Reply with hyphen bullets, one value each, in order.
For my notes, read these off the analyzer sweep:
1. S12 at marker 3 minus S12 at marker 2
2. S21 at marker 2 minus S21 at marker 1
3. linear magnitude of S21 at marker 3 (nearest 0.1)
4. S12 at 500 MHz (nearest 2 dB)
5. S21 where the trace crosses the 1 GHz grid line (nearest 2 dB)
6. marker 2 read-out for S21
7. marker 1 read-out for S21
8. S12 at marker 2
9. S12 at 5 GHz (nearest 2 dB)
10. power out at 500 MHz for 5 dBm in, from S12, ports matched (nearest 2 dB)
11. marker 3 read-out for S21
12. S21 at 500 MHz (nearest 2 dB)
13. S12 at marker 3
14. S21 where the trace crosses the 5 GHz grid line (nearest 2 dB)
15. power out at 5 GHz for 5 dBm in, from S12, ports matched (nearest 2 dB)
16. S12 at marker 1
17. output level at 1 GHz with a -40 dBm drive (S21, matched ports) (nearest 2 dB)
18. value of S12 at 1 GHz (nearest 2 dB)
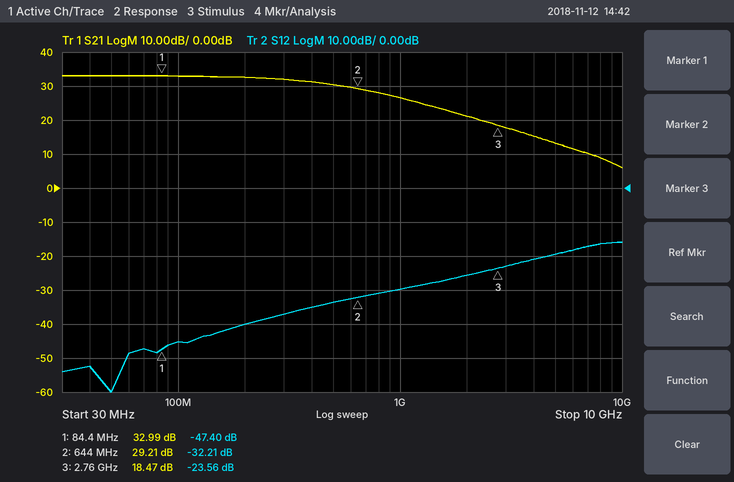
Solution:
- 8.65 dB
- -3.78 dB
- 8.4
- -34 dB
- 26 dB
- 29.21 dB
- 32.99 dB
- -32.21 dB
- -20 dB
- -28 dBm
- 18.47 dB
- 30 dB
- -23.56 dB
- 14 dB
- -14 dBm
- -47.40 dB
- -14 dBm
- -30 dB
